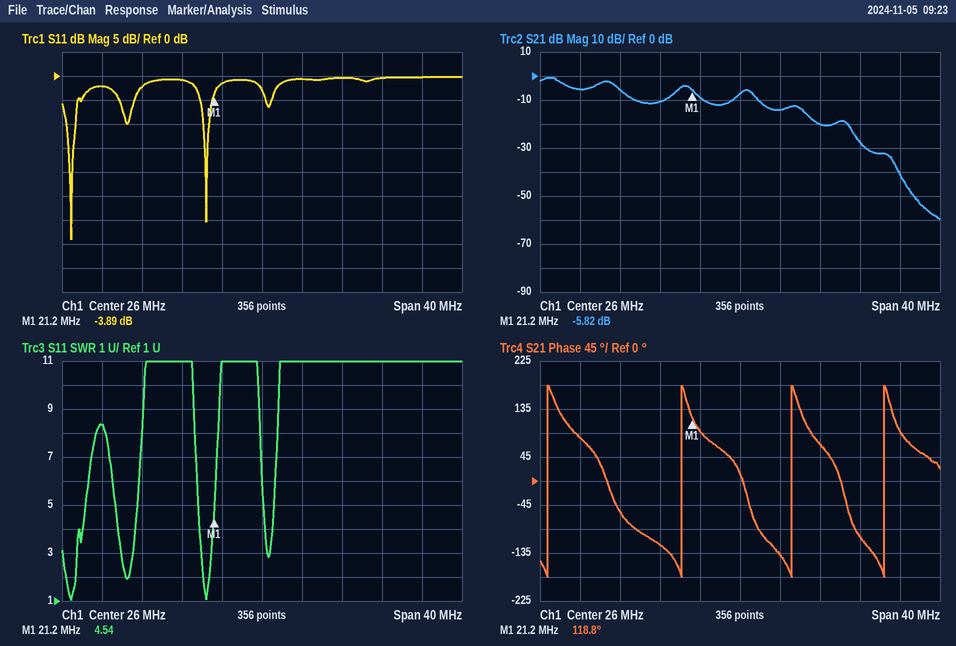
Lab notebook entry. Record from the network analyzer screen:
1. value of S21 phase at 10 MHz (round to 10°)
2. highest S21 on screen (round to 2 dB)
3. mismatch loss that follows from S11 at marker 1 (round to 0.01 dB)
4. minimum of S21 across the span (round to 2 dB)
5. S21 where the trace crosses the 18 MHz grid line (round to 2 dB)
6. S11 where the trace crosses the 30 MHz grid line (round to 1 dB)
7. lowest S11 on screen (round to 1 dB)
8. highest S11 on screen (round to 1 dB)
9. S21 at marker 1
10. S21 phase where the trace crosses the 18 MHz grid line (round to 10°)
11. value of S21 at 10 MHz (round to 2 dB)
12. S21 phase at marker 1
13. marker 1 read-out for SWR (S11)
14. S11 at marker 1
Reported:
80°
0 dB
2.28 dB
-60 dB
-10 dB
-1 dB
-34 dB
0 dB
-5.82 dB
-120°
-6 dB
118.8°
4.54
-3.89 dB
